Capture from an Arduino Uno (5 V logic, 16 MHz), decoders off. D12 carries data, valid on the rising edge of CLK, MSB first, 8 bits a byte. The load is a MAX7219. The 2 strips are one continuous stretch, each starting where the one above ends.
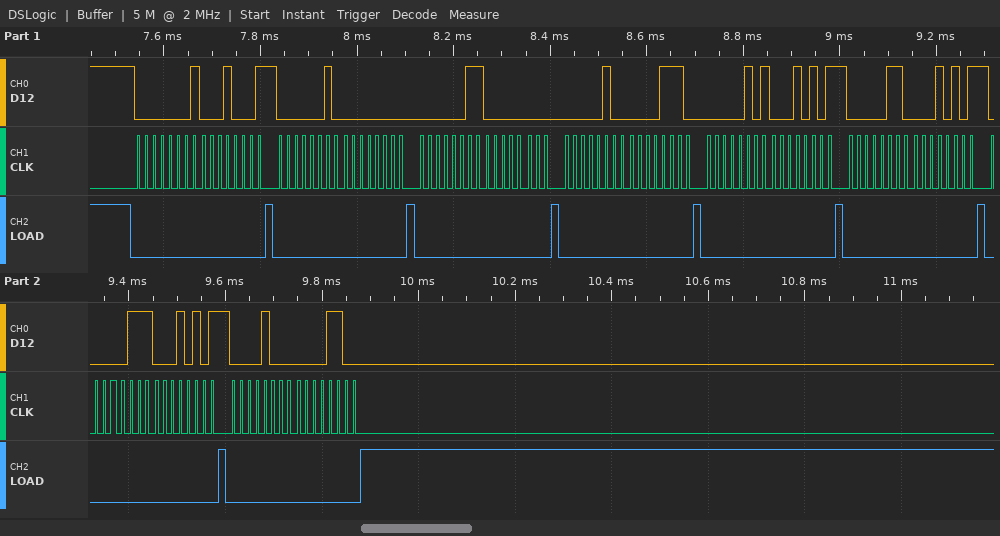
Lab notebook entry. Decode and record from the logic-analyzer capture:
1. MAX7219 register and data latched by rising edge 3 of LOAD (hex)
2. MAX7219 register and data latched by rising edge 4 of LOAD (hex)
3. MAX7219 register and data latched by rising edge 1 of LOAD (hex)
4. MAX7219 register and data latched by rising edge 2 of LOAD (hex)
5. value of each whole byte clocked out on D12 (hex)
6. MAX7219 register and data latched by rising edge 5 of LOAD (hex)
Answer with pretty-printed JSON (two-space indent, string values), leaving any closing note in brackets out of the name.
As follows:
{
  "MAX7219 register and data latched by rising edge 3 of LOAD": "register 0x3, data 0x00",
  "MAX7219 register and data latched by rising edge 4 of LOAD": "register 0x4, data 0x0E",
  "MAX7219 register and data latched by rising edge 1 of LOAD": "register 0x1, data 0x11",
  "MAX7219 register and data latched by rising edge 2 of LOAD": "register 0x2, data 0x00",
  "value of each whole byte clocked out on D12": "0x01 0x11 0x02 0x00 0x03 0x00 0x04 0x0E 0x05 0x15 0x06 0x15 0x07 0x15 0x08 0x0C",
  "MAX7219 register and data latched by rising edge 5 of LOAD": "register 0x5, data 0x15"
}
